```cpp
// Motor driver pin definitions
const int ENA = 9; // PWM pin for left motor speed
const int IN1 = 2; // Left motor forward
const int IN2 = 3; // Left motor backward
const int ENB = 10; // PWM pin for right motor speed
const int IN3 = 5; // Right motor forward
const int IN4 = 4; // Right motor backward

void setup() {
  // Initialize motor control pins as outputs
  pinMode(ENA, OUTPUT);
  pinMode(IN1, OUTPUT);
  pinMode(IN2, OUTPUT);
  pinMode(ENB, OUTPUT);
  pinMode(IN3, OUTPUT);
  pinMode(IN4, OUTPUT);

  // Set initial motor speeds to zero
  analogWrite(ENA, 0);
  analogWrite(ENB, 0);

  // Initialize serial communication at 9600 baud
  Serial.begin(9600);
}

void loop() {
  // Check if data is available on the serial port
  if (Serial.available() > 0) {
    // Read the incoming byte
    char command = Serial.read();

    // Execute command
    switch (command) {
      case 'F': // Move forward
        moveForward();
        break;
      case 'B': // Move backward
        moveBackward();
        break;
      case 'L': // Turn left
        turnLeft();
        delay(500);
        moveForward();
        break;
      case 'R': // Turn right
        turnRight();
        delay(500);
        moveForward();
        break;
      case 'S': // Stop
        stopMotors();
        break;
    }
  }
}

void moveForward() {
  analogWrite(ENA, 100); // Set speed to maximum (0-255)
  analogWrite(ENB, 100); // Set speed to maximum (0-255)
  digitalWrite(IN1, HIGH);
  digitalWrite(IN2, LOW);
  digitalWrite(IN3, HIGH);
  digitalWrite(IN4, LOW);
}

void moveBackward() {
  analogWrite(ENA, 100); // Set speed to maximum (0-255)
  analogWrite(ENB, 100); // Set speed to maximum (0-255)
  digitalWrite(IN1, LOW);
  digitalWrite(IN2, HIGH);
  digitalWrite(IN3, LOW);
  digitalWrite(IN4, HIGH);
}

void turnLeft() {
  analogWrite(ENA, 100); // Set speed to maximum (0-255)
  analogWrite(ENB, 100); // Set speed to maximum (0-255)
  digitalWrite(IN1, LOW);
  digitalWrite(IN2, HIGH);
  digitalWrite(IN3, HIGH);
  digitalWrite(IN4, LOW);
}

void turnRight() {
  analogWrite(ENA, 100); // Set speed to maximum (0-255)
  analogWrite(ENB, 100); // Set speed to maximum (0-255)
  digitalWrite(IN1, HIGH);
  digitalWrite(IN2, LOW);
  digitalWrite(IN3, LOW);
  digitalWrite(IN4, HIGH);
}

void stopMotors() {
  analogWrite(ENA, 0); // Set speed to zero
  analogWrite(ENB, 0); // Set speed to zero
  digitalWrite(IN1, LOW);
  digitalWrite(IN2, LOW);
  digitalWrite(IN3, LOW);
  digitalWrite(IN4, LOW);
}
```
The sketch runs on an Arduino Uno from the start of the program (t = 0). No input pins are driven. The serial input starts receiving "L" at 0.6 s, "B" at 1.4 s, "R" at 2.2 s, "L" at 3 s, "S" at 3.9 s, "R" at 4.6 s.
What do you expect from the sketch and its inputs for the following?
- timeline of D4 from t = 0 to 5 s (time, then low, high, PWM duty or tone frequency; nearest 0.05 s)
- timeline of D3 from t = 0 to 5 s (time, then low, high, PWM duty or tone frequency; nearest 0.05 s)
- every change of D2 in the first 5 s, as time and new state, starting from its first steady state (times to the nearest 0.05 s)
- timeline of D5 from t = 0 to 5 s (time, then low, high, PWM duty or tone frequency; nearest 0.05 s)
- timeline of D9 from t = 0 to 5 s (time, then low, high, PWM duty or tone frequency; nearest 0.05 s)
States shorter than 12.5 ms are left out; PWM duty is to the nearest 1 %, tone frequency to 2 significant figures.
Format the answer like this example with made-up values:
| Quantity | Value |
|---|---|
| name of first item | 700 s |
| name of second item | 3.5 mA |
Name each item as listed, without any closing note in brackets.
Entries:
| Quantity | Value |
|---|---|
| timeline of D4 from t = 0 to 5 s | 0 s low; 1.4 s high; 2.7 s low; 4.6 s high |
| timeline of D3 from t = 0 to 5 s | 0 s low; 0.6 s high; 1.1 s low; 1.4 s high; 2.2 s low; 3 s high; 3.5 s low |
| every change of D2 in the first 5 s, as time and new state, starting from its first steady state | 0 s low; 1.1 s high; 1.4 s low; 2.2 s high; 3 s low; 3.5 s high; 3.9 s low; 4.6 s high |
| timeline of D5 from t = 0 to 5 s | 0 s low; 0.6 s high; 1.4 s low; 2.7 s high; 3.9 s low |
| timeline of D9 from t = 0 to 5 s | 0 s low; 0.6 s PWM 39 %; 3.9 s low; 4.6 s PWM 39 % |
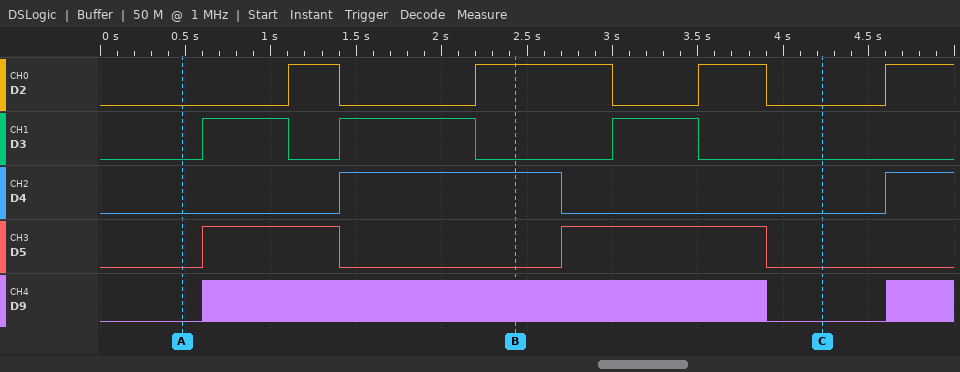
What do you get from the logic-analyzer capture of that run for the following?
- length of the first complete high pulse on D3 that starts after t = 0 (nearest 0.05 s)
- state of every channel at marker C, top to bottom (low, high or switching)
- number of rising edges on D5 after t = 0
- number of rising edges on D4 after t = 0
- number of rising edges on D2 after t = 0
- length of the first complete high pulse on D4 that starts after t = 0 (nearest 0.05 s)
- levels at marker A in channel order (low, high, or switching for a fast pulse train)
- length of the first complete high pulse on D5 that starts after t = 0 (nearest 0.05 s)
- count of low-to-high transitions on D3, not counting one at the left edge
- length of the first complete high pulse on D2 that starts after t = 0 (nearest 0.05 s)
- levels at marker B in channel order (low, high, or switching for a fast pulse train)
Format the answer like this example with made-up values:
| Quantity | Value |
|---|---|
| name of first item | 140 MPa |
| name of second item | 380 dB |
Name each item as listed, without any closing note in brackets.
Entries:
| Quantity | Value |
|---|---|
| length of the first complete high pulse on D3 that starts after t = 0 | 0.50 s |
| state of every channel at marker C, top to bottom | D2 low, D3 low, D4 low, D5 low, D9 low |
| number of rising edges on D5 after t = 0 | 2 |
| number of rising edges on D4 after t = 0 | 2 |
| number of rising edges on D2 after t = 0 | 4 |
| length of the first complete high pulse on D4 that starts after t = 0 | 1.30 s |
| levels at marker A in channel order | D2 low, D3 low, D4 low, D5 low, D9 low |
| length of the first complete high pulse on D5 that starts after t = 0 | 0.80 s |
| count of low-to-high transitions on D3, not counting one at the left edge | 3 |
| length of the first complete high pulse on D2 that starts after t = 0 | 0.30 s |
| levels at marker B in channel order | D2 high, D3 low, D4 high, D5 low, D9 switching |
